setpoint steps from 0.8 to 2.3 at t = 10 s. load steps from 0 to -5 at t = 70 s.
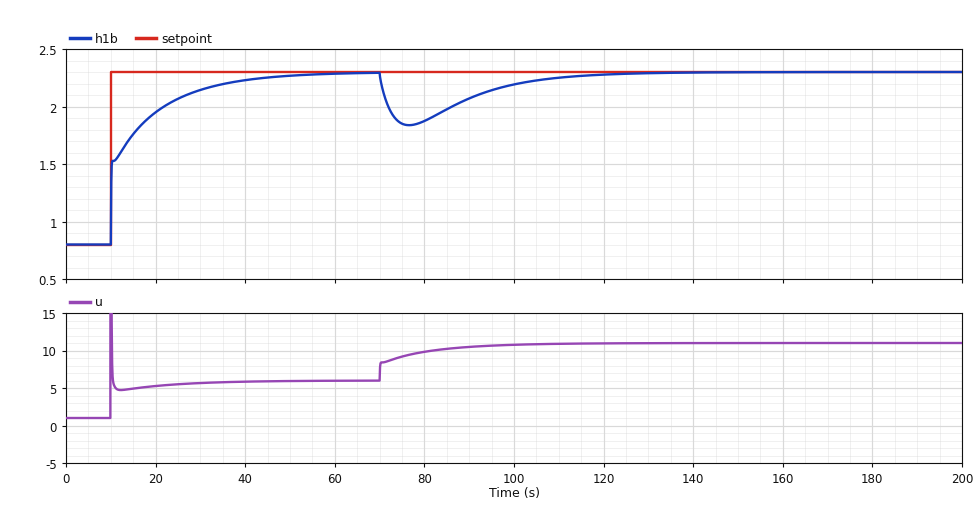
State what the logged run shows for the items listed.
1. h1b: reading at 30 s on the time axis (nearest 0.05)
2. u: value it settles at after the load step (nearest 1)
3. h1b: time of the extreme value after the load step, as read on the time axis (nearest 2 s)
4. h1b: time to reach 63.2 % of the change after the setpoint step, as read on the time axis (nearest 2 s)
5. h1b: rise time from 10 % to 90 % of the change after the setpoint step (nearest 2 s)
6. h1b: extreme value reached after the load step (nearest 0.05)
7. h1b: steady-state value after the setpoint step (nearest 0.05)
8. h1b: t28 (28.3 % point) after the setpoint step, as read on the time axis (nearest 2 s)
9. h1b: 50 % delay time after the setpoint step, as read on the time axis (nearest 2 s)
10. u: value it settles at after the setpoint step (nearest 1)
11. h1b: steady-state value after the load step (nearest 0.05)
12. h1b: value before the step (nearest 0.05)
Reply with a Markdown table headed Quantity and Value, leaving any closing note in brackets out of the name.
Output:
| Quantity | Value |
|---|---|
| h1b: reading at 30 s on the time axis | 2.15 |
| u: value it settles at after the load step | 11 |
| h1b: time of the extreme value after the load step, as read on the time axis | 76 s |
| h1b: time to reach 63.2 % of the change after the setpoint step, as read on the time axis | 14 s |
| h1b: rise time from 10 % to 90 % of the change after the setpoint step | 20 s |
| h1b: extreme value reached after the load step | 1.85 |
| h1b: steady-state value after the setpoint step | 2.30 |
| h1b: t28 (28.3 % point) after the setpoint step, as read on the time axis | 10 s |
| h1b: 50 % delay time after the setpoint step, as read on the time axis | 12 s |
| u: value it settles at after the setpoint step | 6 |
| h1b: steady-state value after the load step | 2.30 |
| h1b: value before the step | 0.80 |
